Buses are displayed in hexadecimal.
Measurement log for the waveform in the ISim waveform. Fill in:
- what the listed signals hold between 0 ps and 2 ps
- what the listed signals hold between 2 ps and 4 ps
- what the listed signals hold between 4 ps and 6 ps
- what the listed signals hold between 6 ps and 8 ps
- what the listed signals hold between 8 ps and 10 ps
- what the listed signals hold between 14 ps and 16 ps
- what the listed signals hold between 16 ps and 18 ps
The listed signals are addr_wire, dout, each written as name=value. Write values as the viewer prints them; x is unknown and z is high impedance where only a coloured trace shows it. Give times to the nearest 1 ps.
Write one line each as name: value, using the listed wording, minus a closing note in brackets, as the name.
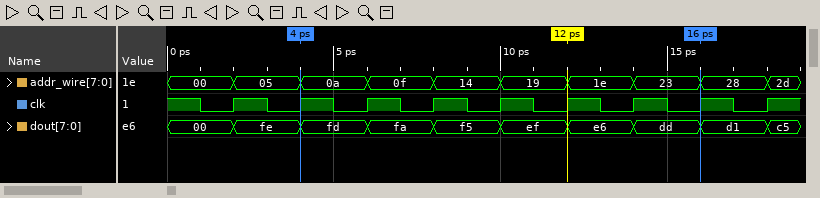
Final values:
what the listed signals hold between 0 ps and 2 ps: addr_wire=00, dout=00
what the listed signals hold between 2 ps and 4 ps: addr_wire=05, dout=fe
what the listed signals hold between 4 ps and 6 ps: addr_wire=0a, dout=fd
what the listed signals hold between 6 ps and 8 ps: addr_wire=0f, dout=fa
what the listed signals hold between 8 ps and 10 ps: addr_wire=14, dout=f5
what the listed signals hold between 14 ps and 16 ps: addr_wire=23, dout=dd
what the listed signals hold between 16 ps and 18 ps: addr_wire=28, dout=d1
